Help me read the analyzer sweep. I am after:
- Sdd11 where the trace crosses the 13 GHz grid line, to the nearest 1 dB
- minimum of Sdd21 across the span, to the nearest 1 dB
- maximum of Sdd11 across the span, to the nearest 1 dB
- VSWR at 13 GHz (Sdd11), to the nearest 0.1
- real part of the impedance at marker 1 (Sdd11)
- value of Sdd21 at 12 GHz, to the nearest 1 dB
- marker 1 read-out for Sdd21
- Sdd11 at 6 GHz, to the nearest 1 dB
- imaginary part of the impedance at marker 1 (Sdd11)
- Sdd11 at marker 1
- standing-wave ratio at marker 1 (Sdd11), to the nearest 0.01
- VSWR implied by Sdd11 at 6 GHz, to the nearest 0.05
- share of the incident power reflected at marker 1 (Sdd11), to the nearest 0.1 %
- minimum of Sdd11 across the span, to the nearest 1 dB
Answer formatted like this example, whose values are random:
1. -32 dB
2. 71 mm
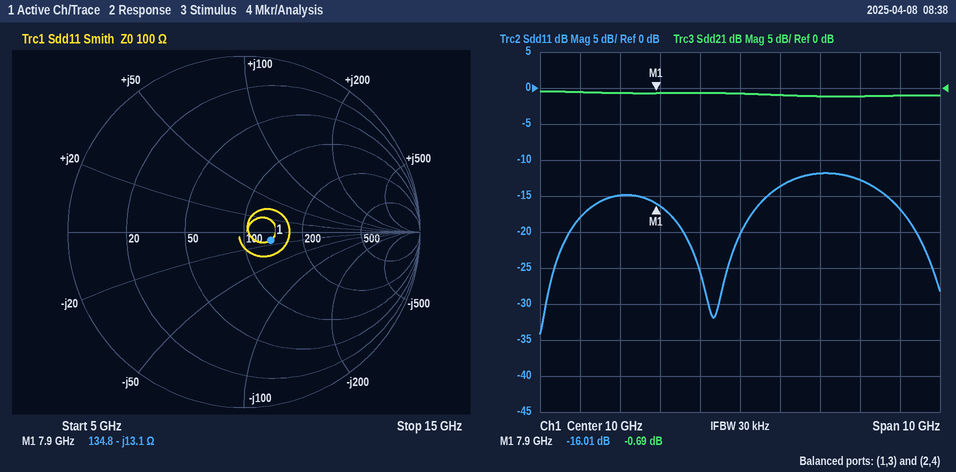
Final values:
1. -13 dB
2. -1 dB
3. -12 dB
4. 1.6
5. 134.8 Ω
6. -1 dB
7. -0.69 dB
8. -18 dB
9. -13.1 Ω
10. -16.01 dB
11. 1.38
12. 1.30
13. 2.5 %
14. -34 dB
